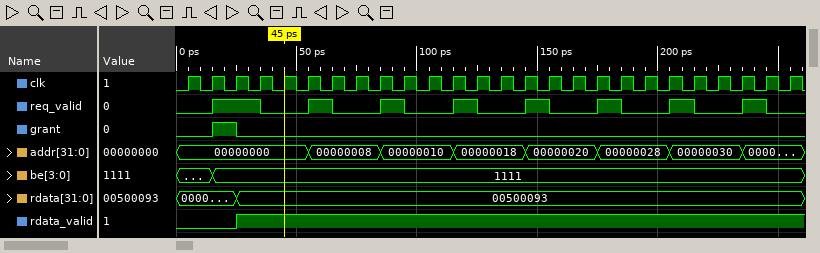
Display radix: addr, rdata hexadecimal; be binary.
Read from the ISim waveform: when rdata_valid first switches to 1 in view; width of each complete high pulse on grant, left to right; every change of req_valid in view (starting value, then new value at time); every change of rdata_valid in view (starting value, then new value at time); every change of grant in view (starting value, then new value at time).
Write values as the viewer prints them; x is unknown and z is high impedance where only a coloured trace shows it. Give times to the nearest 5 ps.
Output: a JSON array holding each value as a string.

["25 ps", "10 ps", "0, 1 at 15 ps, 0 at 35 ps, 1 at 55 ps, 0 at 65 ps, 1 at 85 ps, 0 at 95 ps, 1 at 115 ps, 0 at 125 ps, 1 at 145 ps, 0 at 155 ps, 1 at 175 ps, 0 at 185 ps, 1 at 205 ps, 0 at 215 ps, 1 at 235 ps, 0 at 245 ps", "0, 1 at 25 ps", "0, 1 at 15 ps, 0 at 25 ps"]
